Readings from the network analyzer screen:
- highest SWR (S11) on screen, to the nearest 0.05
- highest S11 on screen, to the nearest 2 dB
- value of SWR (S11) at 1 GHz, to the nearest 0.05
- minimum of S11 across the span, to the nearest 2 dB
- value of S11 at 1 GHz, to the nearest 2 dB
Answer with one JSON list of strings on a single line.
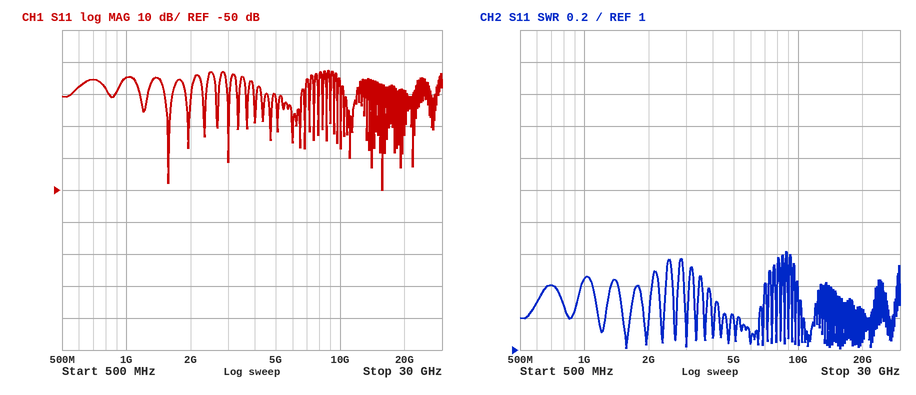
["1.60", "-12 dB", "1.45", "-50 dB", "-14 dB"]
